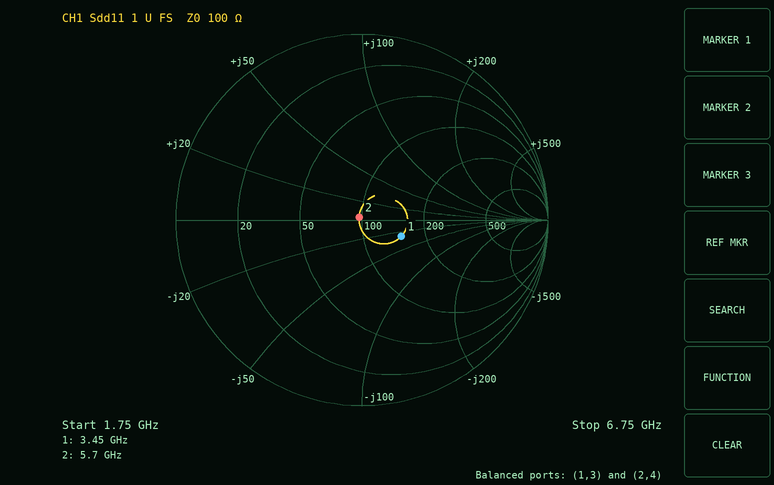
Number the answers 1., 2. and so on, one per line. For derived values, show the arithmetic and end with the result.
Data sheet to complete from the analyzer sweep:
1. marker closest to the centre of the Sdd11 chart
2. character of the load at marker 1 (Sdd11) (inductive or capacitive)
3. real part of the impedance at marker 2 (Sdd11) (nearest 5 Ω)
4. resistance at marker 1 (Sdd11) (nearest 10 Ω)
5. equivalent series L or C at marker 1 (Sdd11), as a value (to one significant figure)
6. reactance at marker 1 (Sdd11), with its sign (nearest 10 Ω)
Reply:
1. marker 2
2. capacitive
3. 95 Ω
4. 150 Ω
5. C = 1/(2π × 3.45 GHz × 30 Ω) ≈ 2 pF
6. -30 Ω
